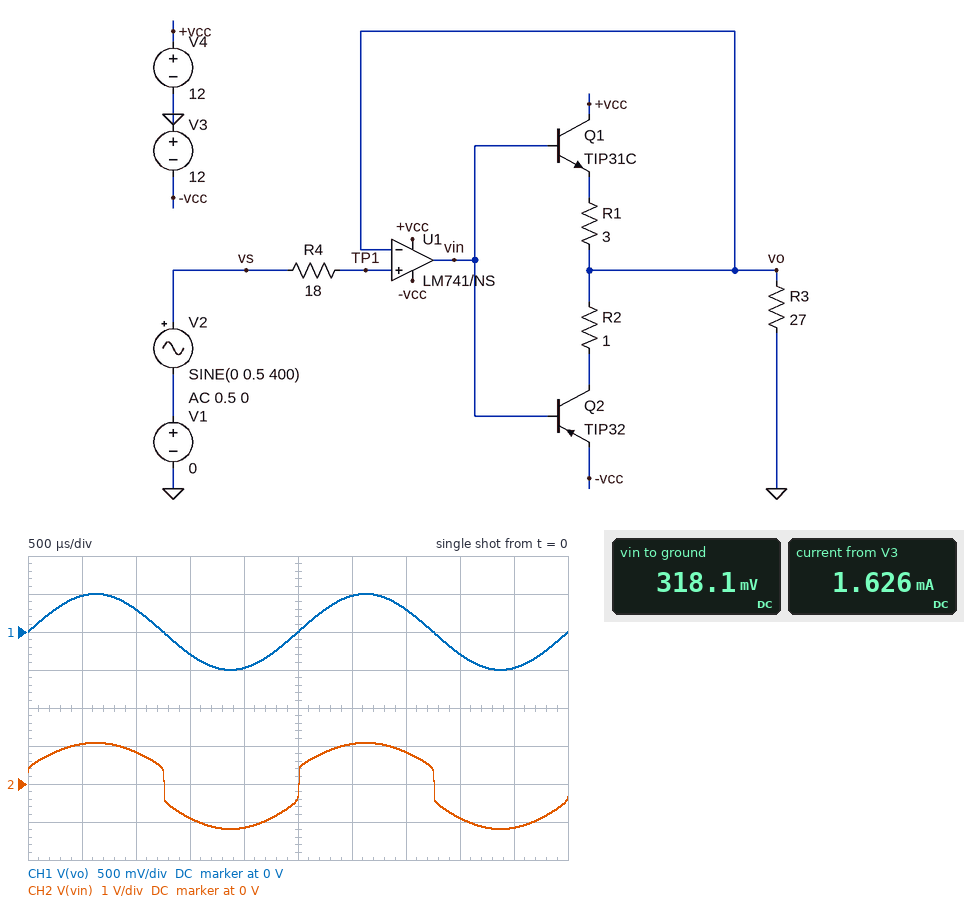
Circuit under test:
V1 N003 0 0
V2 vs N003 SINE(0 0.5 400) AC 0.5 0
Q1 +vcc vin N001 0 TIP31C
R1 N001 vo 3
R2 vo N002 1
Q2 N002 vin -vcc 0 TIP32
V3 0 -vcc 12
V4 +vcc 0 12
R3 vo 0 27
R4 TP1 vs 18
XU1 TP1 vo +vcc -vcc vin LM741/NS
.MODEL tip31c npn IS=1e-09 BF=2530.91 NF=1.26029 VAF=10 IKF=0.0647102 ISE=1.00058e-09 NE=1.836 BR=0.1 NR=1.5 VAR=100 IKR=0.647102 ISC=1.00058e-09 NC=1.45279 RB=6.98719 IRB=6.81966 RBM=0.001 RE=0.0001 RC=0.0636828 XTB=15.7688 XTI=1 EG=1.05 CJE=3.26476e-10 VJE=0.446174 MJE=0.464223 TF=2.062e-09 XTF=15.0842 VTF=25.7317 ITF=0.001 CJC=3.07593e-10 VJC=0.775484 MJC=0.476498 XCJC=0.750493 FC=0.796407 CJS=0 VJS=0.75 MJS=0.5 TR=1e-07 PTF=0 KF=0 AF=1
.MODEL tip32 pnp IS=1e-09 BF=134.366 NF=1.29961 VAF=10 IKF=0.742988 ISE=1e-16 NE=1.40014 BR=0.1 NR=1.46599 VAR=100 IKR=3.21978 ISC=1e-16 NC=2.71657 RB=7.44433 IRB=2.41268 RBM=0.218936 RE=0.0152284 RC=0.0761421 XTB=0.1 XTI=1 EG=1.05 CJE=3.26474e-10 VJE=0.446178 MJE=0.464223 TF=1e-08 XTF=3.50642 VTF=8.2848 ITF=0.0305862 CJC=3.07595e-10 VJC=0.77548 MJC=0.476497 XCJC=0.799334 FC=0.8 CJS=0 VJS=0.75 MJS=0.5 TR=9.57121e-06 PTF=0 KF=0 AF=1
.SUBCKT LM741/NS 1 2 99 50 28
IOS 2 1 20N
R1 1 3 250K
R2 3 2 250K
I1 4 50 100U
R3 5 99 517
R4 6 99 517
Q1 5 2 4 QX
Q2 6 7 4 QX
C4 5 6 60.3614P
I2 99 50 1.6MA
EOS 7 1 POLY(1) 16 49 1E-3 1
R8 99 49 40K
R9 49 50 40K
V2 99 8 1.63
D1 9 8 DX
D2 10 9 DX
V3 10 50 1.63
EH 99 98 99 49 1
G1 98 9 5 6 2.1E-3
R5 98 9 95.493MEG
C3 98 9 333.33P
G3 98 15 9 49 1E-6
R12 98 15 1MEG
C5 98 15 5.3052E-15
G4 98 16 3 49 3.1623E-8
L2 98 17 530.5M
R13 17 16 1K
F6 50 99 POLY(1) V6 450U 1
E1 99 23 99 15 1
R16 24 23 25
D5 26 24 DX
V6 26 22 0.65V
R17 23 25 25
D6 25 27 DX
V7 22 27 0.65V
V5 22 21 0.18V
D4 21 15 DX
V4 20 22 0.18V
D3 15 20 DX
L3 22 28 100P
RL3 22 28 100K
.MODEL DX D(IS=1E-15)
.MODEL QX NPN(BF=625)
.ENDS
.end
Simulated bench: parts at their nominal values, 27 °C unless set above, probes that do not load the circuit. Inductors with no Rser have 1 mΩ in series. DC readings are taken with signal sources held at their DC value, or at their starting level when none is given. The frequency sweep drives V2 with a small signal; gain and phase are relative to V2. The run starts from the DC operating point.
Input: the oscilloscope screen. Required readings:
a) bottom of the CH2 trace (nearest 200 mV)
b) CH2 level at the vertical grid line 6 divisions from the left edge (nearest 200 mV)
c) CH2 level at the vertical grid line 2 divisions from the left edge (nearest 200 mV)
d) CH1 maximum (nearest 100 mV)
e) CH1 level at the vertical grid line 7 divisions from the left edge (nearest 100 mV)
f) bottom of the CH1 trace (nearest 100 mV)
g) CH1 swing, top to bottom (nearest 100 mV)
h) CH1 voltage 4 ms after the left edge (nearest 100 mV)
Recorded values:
-1.2 V
1.0 V
800 mV
500 mV
300 mV
-500 mV
1.0 V
-300 mV
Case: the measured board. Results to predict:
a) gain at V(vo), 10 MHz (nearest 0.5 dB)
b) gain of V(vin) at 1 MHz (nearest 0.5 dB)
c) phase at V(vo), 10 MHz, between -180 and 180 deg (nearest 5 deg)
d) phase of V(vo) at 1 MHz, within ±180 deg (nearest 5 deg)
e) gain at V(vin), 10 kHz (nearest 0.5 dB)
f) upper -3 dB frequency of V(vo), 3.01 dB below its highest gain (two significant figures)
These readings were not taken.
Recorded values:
-51.0 dB
-4.5 dB
-165 deg
-80 deg
30.0 dB
27 kHz
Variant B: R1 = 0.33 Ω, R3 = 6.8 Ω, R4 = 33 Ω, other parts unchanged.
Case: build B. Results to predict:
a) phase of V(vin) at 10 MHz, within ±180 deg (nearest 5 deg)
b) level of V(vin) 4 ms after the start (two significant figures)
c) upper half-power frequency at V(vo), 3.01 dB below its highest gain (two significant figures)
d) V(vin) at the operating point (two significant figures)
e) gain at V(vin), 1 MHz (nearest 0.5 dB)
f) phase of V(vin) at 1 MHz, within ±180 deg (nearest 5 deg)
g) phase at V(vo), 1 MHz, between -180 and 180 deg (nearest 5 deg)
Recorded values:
150 deg
-960 mV
30 kHz
360 mV
-5.0 dB
-160 deg
-110 deg
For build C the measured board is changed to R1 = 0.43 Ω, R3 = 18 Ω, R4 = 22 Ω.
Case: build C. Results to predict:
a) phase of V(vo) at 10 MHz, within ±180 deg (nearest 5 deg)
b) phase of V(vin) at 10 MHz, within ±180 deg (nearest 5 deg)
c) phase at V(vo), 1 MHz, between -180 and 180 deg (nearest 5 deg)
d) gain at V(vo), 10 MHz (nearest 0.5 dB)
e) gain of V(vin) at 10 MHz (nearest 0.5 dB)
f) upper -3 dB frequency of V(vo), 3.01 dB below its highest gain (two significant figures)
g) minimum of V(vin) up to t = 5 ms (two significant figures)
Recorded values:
-160 deg
160 deg
-85 deg
-54.0 dB
-50.0 dB
28 kHz
-1.3 V
